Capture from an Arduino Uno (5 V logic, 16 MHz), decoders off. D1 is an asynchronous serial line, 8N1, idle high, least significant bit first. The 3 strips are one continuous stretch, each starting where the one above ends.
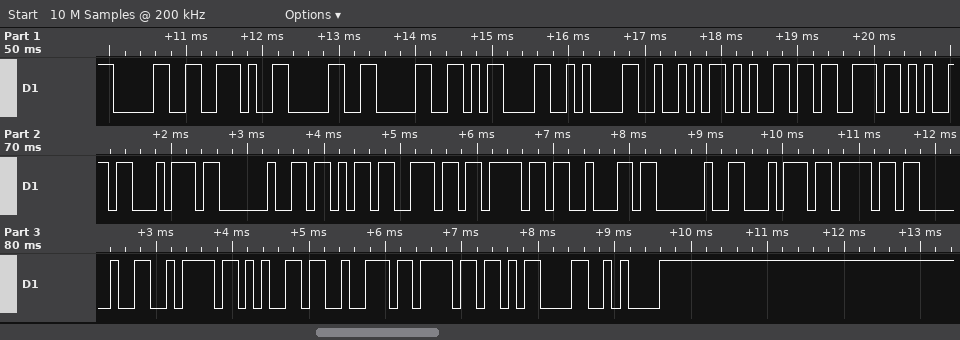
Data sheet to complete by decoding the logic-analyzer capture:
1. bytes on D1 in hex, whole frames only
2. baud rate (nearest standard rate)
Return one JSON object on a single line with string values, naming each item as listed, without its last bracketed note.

{"bytes on D1 in hex, whole frames only": "30 2E 30 30 0D 0A 52 65 73 65 74 20 6B 6E 6F 62 20 74 6F 20 7A 65 72 6F 0D 0A", "baud rate": "9600 baud"}
